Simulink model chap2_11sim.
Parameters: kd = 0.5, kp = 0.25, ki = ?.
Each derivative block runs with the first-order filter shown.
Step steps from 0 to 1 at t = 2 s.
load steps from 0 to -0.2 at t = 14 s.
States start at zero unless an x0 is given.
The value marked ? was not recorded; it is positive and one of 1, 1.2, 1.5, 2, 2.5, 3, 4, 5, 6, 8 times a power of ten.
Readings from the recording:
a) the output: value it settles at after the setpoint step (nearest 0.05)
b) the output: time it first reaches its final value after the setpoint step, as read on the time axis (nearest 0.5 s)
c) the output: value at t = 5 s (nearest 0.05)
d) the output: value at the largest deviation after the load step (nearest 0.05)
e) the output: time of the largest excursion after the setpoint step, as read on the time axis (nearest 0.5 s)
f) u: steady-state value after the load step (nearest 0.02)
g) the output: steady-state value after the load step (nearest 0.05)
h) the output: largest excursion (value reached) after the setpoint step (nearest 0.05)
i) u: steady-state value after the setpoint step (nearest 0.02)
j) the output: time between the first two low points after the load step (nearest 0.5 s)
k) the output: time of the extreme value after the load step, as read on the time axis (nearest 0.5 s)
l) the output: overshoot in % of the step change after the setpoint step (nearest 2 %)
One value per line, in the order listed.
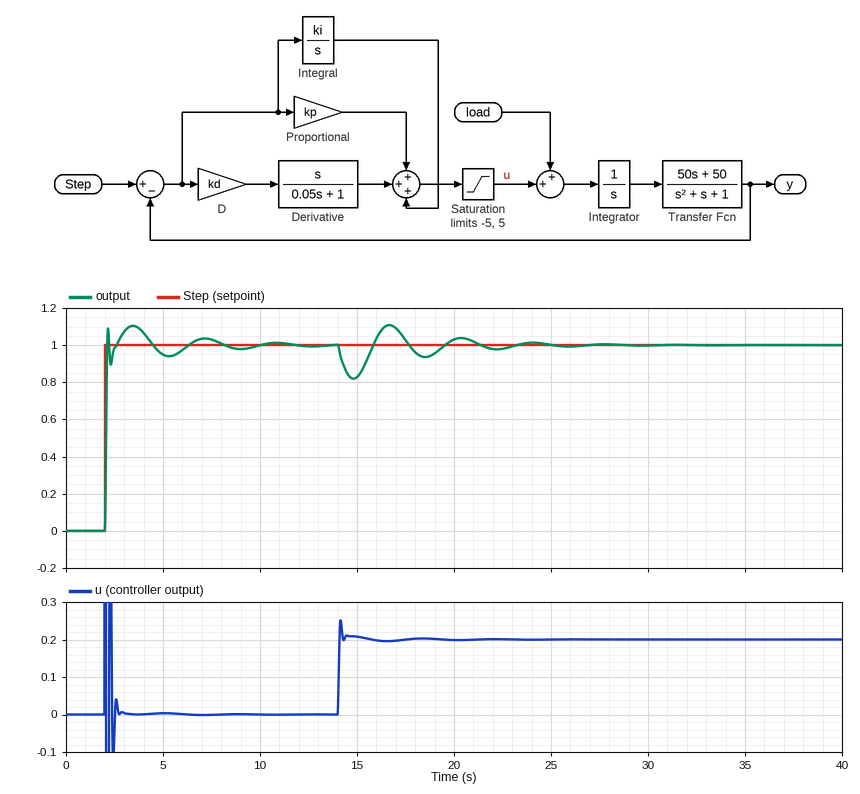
1.00
2.0 s
0.95
0.80
3.5 s
0.20
1.00
1.10
0.00
3.5 s
15.0 s
10 %
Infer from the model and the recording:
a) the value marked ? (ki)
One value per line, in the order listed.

1.5
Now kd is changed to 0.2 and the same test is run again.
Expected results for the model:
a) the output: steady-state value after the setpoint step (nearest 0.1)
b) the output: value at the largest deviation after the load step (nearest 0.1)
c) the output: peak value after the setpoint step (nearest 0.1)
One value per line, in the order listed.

1.0
0.7
1.3
